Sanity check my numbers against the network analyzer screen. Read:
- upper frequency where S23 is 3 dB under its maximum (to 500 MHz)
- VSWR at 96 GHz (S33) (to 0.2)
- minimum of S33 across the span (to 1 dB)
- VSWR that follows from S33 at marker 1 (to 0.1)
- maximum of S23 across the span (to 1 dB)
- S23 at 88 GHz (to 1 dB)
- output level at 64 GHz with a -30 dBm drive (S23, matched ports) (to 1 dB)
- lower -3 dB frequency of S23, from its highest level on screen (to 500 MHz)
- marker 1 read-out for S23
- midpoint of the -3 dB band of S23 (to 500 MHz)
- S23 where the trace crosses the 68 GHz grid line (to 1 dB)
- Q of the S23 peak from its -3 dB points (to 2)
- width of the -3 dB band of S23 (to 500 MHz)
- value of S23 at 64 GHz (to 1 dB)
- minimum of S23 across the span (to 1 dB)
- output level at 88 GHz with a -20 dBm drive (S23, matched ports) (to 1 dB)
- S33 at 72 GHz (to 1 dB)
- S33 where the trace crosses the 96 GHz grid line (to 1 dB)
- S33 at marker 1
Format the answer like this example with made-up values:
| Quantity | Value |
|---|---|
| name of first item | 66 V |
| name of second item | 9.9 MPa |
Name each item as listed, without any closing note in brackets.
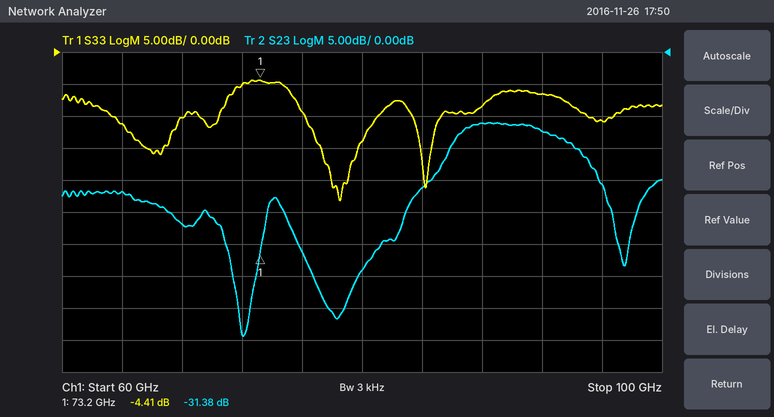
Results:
| Quantity | Value |
|---|---|
| upper frequency where S23 is 3 dB under its maximum | 93.5 GHz |
| VSWR at 96 GHz (S33) | 1.8 |
| minimum of S33 across the span | -23 dB |
| VSWR that follows from S33 at marker 1 | 4.0 |
| maximum of S23 across the span | -11 dB |
| S23 at 88 GHz | -11 dB |
| output level at 64 GHz with a -30 dBm drive (S23, matched ports) | -52 dBm |
| lower -3 dB frequency of S23, from its highest level on screen | 86.0 GHz |
| marker 1 read-out for S23 | -31.38 dB |
| midpoint of the -3 dB band of S23 | 90.0 GHz |
| S23 where the trace crosses the 68 GHz grid line | -27 dB |
| Q of the S23 peak from its -3 dB points | 12 |
| width of the -3 dB band of S23 | 7.5 GHz |
| value of S23 at 64 GHz | -22 dB |
| minimum of S23 across the span | -44 dB |
| output level at 88 GHz with a -20 dBm drive (S23, matched ports) | -31 dBm |
| S33 at 72 GHz | -5 dB |
| S33 where the trace crosses the 96 GHz grid line | -11 dB |
| S33 at marker 1 | -4.41 dB |
